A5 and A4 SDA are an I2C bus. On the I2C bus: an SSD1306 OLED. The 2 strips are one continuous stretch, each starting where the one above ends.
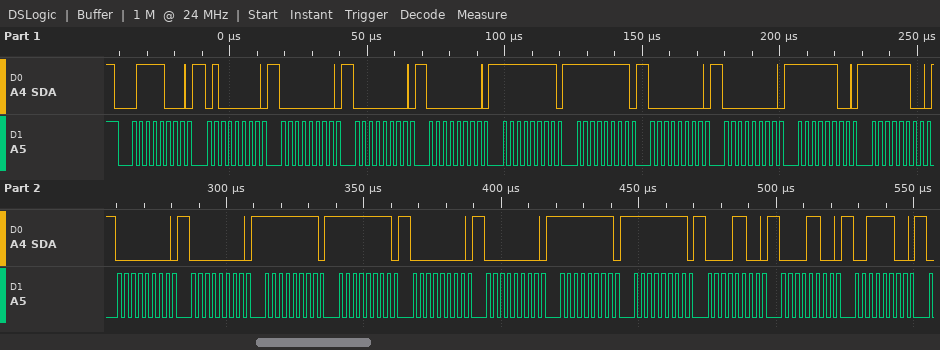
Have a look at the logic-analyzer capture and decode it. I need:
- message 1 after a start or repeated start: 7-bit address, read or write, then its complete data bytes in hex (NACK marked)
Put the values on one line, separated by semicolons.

0x3C write: 40 00 00 00 FF FF 00 00 FC FC 00 00 FF FF 00 00 FF FF 0C 0C 3C
